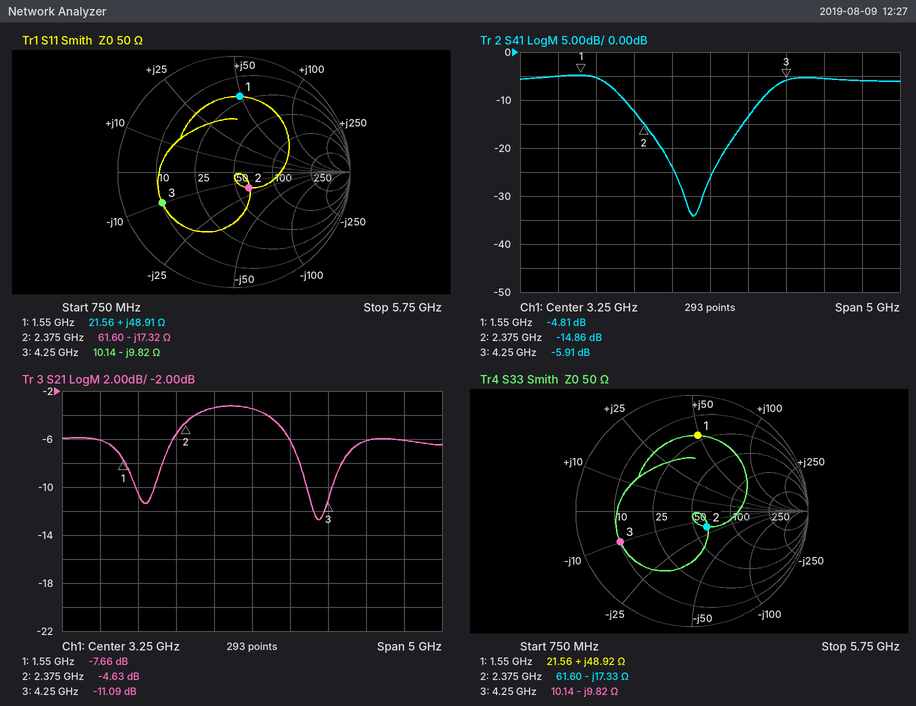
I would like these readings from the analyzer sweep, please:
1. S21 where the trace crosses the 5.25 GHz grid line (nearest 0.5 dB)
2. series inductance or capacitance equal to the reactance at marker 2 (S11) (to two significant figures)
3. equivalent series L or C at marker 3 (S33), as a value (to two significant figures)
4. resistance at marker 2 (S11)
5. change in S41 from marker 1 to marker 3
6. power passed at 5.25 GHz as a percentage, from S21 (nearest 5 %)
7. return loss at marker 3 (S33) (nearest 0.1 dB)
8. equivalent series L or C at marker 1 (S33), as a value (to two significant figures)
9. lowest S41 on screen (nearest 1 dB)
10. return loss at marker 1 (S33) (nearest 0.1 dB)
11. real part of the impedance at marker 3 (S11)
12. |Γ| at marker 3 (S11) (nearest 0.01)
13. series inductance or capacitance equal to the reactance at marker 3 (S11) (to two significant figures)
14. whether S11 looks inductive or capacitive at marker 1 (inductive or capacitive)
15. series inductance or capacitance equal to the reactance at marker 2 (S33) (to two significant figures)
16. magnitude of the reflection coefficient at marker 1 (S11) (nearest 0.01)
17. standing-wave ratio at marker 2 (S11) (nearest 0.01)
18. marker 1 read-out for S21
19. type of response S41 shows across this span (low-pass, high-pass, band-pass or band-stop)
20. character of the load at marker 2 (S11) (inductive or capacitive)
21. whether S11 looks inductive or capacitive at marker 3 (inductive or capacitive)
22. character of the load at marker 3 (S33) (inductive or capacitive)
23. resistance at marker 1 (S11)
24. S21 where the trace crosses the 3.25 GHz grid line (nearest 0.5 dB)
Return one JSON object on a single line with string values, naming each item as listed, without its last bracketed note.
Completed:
{"S21 where the trace crosses the 5.25 GHz grid line": "-6.0 dB", "series inductance or capacitance equal to the reactance at marker 2 (S11)": "3.9 pF", "equivalent series L or C at marker 3 (S33), as a value": "3.8 pF", "resistance at marker 2": "61.60 Ω", "change in S41 from marker 1 to marker 3": "-1.10 dB", "power passed at 5.25 GHz as a percentage, from S21": "25 %", "return loss at marker 3 (S33)": "3.4 dB", "equivalent series L or C at marker 1 (S33), as a value": "5.0 nH", "lowest S41 on screen": "-34 dB", "return loss at marker 1 (S33)": "3.7 dB", "real part of the impedance at marker 3": "10.14 Ω", "|Γ| at marker 3 (S11)": "0.67", "series inductance or capacitance equal to the reactance at marker 3 (S11)": "3.8 pF", "whether S11 looks inductive or capacitive at marker 1": "inductive", "series inductance or capacitance equal to the reactance at marker 2 (S33)": "3.9 pF", "magnitude of the reflection coefficient at marker 1 (S11)": "0.65", "standing-wave ratio at marker 2 (S11)": "1.45", "marker 1 read-out for S21": "-7.66 dB", "type of response S41 shows across this span": "band-stop", "character of the load at marker 2 (S11)": "capacitive", "whether S11 looks inductive or capacitive at marker 3": "capacitive", "character of the load at marker 3 (S33)": "capacitive", "resistance at marker 1": "21.56 Ω", "S21 where the trace crosses the 3.25 GHz grid line": "-3.5 dB"}
